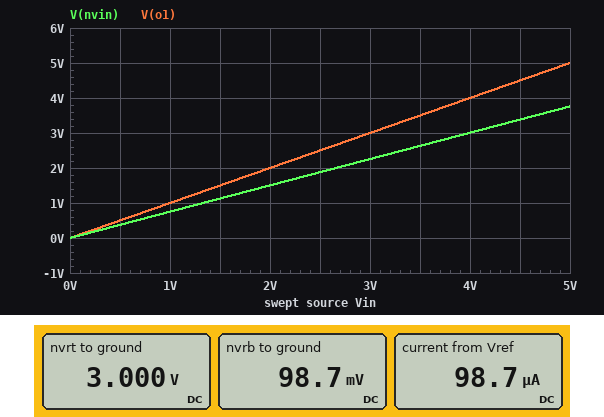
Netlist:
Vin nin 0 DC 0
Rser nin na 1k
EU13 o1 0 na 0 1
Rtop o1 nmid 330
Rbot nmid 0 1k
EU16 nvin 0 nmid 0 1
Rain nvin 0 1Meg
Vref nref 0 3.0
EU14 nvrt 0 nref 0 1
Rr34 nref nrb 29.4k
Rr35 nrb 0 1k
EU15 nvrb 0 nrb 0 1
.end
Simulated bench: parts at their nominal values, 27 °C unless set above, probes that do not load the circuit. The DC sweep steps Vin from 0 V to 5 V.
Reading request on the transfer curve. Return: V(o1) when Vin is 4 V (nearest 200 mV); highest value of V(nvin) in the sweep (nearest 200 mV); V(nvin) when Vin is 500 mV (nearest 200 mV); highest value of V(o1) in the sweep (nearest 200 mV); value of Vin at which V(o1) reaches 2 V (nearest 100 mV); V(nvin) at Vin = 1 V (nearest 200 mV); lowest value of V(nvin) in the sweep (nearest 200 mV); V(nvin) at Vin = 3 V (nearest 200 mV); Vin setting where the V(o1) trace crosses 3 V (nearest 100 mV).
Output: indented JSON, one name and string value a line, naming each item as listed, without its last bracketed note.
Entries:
{
  "V(o1) when Vin is 4 V": "4.0 V",
  "highest value of V(nvin) in the sweep": "3.8 V",
  "V(nvin) when Vin is 500 mV": "400 mV",
  "highest value of V(o1) in the sweep": "5.0 V",
  "value of Vin at which V(o1) reaches 2 V": "2.0 V",
  "V(nvin) at Vin = 1 V": "800 mV",
  "lowest value of V(nvin) in the sweep": "0 V",
  "V(nvin) at Vin = 3 V": "2.2 V",
  "Vin setting where the V(o1) trace crosses 3 V": "3.0 V"
}
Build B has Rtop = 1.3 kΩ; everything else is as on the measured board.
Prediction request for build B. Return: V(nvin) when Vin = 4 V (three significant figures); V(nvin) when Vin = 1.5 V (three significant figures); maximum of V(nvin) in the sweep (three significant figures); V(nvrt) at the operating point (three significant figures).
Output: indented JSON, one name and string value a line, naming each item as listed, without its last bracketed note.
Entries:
{
  "V(nvin) when Vin = 4 V": "1.74 V",
  "V(nvin) when Vin = 1.5 V": "652 mV",
  "maximum of V(nvin) in the sweep": "2.17 V",
  "V(nvrt) at the operating point": "3.00 V"
}
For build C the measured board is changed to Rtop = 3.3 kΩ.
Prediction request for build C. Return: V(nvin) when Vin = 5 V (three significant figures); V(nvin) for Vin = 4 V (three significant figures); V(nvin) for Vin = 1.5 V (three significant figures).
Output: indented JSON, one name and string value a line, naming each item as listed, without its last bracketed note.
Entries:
{
  "V(nvin) when Vin = 5 V": "1.16 V",
  "V(nvin) for Vin = 4 V": "930 mV",
  "V(nvin) for Vin = 1.5 V": "349 mV"
}
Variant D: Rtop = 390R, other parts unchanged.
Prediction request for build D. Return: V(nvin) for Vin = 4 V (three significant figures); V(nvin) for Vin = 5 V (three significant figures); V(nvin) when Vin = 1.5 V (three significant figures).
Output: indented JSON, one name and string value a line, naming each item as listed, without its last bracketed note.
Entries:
{
  "V(nvin) for Vin = 4 V": "2.88 V",
  "V(nvin) for Vin = 5 V": "3.60 V",
  "V(nvin) when Vin = 1.5 V": "1.08 V"
}
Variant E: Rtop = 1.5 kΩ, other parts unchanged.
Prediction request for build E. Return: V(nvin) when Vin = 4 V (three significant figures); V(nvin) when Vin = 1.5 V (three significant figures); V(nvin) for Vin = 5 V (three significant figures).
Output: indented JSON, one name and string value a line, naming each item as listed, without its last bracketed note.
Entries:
{
  "V(nvin) when Vin = 4 V": "1.60 V",
  "V(nvin) when Vin = 1.5 V": "600 mV",
  "V(nvin) for Vin = 5 V": "2.00 V"
}
